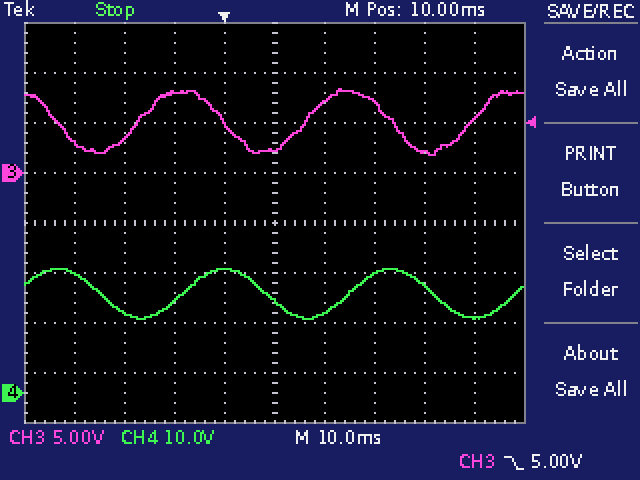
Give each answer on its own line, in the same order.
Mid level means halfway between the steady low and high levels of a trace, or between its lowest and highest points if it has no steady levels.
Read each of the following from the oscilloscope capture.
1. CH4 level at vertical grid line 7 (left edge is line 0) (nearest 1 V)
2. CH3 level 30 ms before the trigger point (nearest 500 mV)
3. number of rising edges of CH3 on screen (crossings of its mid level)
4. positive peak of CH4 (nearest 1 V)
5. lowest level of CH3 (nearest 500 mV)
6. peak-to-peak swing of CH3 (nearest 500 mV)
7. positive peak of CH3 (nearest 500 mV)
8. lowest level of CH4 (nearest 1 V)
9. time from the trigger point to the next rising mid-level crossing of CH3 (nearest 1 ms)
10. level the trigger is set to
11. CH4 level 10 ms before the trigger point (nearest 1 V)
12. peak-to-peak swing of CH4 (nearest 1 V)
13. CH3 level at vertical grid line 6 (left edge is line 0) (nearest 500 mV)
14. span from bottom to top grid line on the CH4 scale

24 V
3.0 V
3
25 V
2.0 V
6.5 V
8.5 V
15 V
16 ms
5.00 V
18 V
10 V
7.0 V
80 V
